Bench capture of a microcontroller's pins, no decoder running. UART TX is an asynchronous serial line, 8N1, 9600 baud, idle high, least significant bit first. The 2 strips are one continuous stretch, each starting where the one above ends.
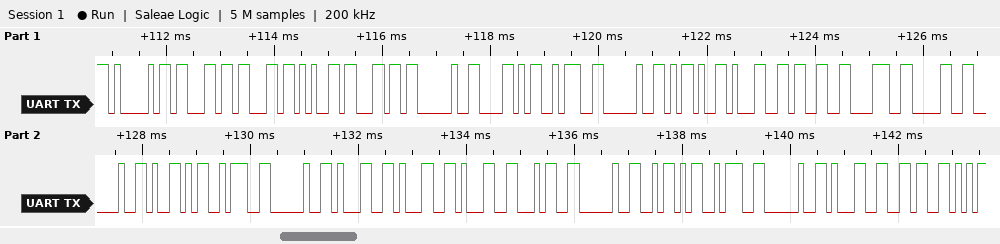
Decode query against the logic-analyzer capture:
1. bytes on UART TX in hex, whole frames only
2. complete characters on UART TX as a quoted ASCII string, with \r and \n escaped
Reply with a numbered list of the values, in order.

1. 0x41 0x63 0x63 0x65 0x6C 0x20 0x58 0x3A 0x20 0x2D 0x31 0x33 0x38 0x30 0x20 0x59 0x3A 0x20 0x31 0x31 0x31 0x34 0x20 0x5A 0x3A 0x20 0x31 0x36
2. "Accel X: -1380 Y: 1114 Z: 16"
